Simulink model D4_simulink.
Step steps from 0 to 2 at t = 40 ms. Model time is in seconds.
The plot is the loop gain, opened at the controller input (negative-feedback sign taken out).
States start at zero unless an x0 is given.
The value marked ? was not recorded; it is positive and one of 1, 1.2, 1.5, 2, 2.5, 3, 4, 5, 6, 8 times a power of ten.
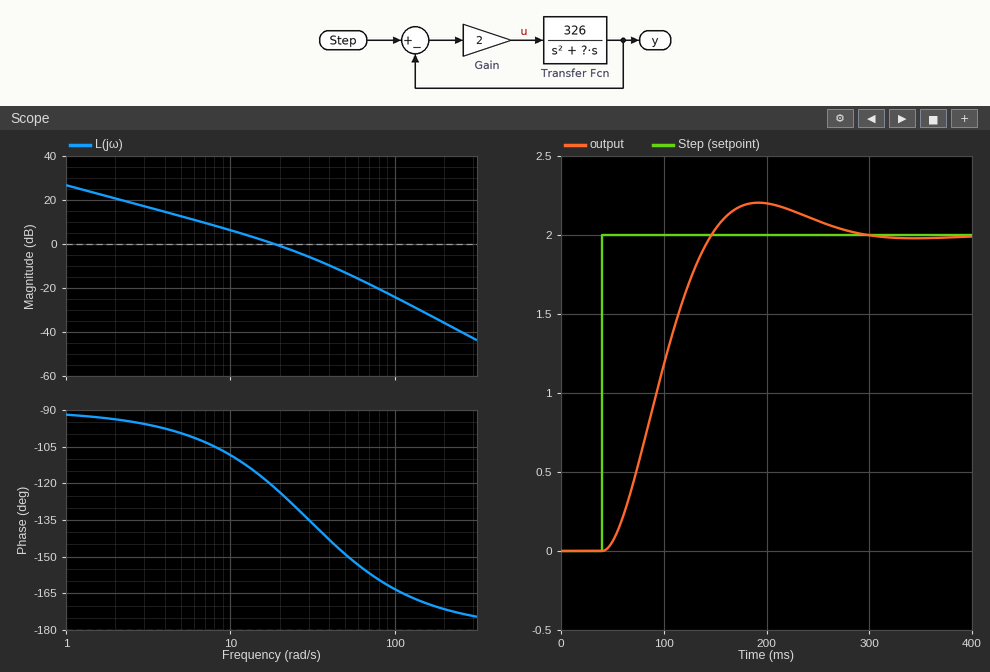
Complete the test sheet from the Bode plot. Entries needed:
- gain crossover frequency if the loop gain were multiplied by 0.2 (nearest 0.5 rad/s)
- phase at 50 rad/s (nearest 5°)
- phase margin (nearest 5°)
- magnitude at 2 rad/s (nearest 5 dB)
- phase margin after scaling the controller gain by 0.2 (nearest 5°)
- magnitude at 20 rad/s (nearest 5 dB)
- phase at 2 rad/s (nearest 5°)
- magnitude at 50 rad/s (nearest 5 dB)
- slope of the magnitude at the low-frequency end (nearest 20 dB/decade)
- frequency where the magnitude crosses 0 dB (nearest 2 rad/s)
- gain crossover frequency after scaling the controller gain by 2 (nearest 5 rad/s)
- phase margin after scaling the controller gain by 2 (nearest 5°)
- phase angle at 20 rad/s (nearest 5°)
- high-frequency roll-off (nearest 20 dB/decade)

4.5 rad/s
-150°
60°
20 dB
80°
0 dB
-95°
-15 dB
-20 dB/decade
18 rad/s
30 rad/s
45°
-125°
-40 dB/decade
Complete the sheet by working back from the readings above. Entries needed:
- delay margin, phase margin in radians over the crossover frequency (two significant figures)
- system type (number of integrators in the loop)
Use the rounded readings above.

0.058 s
1
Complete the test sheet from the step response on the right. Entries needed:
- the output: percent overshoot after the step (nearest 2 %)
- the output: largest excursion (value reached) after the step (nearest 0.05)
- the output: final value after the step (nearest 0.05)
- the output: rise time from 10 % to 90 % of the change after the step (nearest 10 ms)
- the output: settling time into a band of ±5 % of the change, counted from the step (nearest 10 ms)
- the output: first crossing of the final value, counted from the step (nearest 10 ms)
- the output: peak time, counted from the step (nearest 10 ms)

10 %
2.20
2.00
70 ms
210 ms
110 ms
150 ms
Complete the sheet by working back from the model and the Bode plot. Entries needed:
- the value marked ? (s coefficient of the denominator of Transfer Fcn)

30
